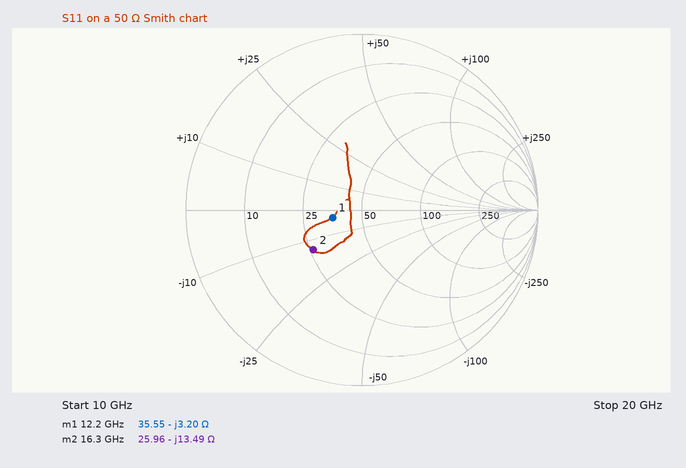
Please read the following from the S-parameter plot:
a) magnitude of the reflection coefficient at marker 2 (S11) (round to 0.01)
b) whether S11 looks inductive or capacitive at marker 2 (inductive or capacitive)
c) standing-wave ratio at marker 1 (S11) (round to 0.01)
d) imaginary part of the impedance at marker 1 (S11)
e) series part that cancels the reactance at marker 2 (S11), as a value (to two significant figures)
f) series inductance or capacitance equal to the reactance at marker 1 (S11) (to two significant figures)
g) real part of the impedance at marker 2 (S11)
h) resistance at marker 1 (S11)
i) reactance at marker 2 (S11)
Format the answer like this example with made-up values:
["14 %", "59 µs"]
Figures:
["0.36", "capacitive", "1.42", "-3.20 Ω", "130 pH", "4.1 pF", "25.96 Ω", "35.55 Ω", "-13.49 Ω"]
